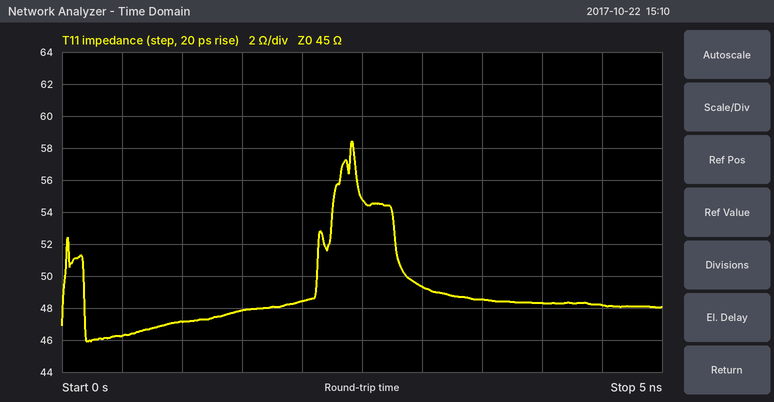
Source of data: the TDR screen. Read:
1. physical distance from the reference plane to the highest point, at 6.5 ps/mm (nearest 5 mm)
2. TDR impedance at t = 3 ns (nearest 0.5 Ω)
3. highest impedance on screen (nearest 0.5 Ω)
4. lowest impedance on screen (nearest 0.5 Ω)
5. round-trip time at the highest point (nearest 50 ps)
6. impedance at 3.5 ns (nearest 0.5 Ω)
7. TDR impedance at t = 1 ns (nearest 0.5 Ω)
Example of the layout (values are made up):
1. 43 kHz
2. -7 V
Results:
1. 185 mm
2. 49.5 Ω
3. 58.5 Ω
4. 46.0 Ω
5. 2.40 ns
6. 48.5 Ω
7. 47.0 Ω
